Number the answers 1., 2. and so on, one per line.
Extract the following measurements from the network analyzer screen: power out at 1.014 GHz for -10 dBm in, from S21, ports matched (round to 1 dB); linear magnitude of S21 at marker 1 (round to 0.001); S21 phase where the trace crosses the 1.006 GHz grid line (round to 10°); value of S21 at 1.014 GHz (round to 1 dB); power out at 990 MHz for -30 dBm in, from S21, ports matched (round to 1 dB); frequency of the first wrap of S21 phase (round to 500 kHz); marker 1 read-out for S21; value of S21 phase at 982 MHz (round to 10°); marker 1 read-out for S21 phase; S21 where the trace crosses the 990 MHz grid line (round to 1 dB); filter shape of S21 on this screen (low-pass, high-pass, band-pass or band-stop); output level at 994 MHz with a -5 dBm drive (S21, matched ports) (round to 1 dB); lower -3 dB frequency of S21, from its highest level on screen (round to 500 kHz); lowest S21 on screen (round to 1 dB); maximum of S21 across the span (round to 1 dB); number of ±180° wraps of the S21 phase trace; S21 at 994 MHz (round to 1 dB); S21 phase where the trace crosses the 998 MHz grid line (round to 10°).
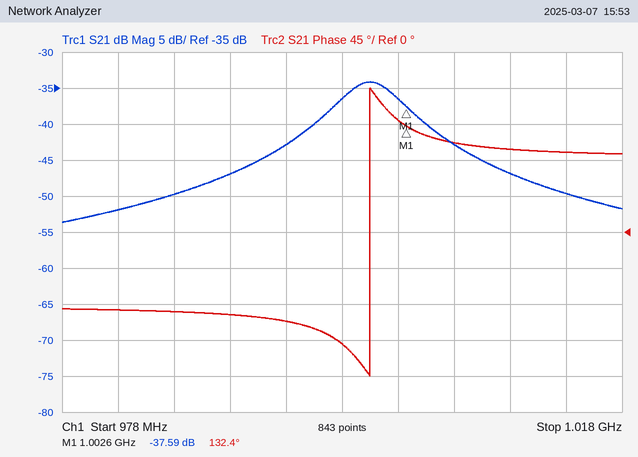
1. -60 dBm
2. 0.013
3. 110°
4. -50 dB
5. -77 dBm
6. 1.0000 GHz
7. -37.59 dB
8. -100°
9. 132.4°
10. -47 dB
11. band-pass
12. -48 dBm
13. 997.5 MHz
14. -54 dB
15. -34 dB
16. 1
17. -43 dB
18. -140°
